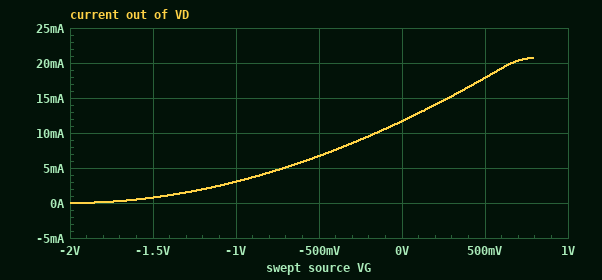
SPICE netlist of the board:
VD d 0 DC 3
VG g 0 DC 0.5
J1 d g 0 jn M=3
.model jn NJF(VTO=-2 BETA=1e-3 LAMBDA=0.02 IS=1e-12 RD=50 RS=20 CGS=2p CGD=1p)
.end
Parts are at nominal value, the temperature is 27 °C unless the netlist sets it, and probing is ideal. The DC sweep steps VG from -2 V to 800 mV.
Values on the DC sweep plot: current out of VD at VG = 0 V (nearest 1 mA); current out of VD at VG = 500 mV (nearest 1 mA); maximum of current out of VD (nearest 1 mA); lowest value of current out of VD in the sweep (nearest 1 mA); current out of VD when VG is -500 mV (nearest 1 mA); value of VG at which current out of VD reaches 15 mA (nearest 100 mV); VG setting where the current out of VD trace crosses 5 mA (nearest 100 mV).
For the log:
12 mA
18 mA
21 mA
0 A
7 mA
300 mV
-700 mV
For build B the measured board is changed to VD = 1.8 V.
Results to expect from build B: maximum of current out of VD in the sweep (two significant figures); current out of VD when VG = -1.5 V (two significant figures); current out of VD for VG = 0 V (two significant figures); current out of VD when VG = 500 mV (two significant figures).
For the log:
16 mA
760 µA
11 mA
15 mA
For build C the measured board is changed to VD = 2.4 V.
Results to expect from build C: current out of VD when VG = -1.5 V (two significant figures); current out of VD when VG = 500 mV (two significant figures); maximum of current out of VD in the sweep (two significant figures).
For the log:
770 µA
17 mA
19 mA
